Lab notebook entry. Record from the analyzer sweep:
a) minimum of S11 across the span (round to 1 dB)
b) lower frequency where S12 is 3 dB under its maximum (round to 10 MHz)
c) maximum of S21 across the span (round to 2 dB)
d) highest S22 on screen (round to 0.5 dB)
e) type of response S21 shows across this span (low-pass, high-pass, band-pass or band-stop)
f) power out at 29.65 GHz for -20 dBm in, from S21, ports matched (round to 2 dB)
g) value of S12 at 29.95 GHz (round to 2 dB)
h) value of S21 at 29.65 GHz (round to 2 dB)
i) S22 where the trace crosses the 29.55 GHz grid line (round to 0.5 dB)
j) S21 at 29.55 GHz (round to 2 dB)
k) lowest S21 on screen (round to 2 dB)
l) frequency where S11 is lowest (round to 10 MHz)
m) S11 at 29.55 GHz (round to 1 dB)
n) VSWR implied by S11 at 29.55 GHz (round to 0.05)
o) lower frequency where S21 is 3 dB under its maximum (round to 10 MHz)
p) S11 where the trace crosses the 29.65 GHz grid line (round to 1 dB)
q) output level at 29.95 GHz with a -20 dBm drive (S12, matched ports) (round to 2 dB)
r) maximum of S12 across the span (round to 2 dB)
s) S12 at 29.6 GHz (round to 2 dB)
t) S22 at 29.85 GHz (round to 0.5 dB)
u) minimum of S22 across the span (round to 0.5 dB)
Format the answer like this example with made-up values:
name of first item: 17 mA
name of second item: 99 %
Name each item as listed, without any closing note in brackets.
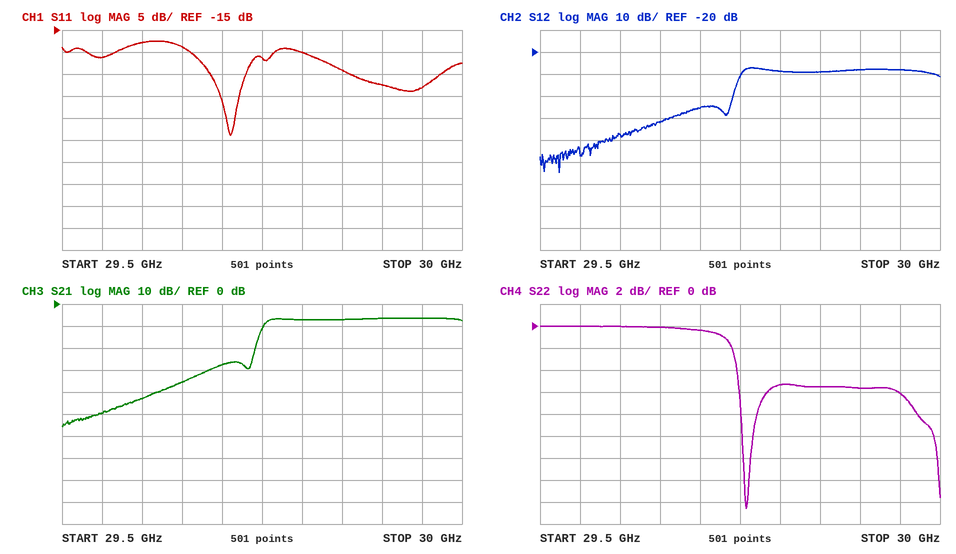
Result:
minimum of S11 across the span: -39 dB
lower frequency where S12 is 3 dB under its maximum: 29.75 GHz
maximum of S21 across the span: -6 dB
highest S22 on screen: 0.0 dB
type of response S21 shows across this span: high-pass
power out at 29.65 GHz for -20 dBm in, from S21, ports matched: -56 dBm
value of S12 at 29.95 GHz: -28 dB
value of S21 at 29.65 GHz: -36 dB
S22 where the trace crosses the 29.55 GHz grid line: 0.0 dB
S21 at 29.55 GHz: -50 dB
lowest S21 on screen: -56 dB
frequency where S11 is lowest: 29.71 GHz
S11 at 29.55 GHz: -21 dB
VSWR implied by S11 at 29.55 GHz: 1.20
lower frequency where S21 is 3 dB under its maximum: 29.75 GHz
S11 where the trace crosses the 29.65 GHz grid line: -19 dB
output level at 29.95 GHz with a -20 dBm drive (S12, matched ports): -48 dBm
maximum of S12 across the span: -28 dB
S12 at 29.6 GHz: -58 dB
S22 at 29.85 GHz: -5.5 dB
minimum of S22 across the span: -16.5 dB
